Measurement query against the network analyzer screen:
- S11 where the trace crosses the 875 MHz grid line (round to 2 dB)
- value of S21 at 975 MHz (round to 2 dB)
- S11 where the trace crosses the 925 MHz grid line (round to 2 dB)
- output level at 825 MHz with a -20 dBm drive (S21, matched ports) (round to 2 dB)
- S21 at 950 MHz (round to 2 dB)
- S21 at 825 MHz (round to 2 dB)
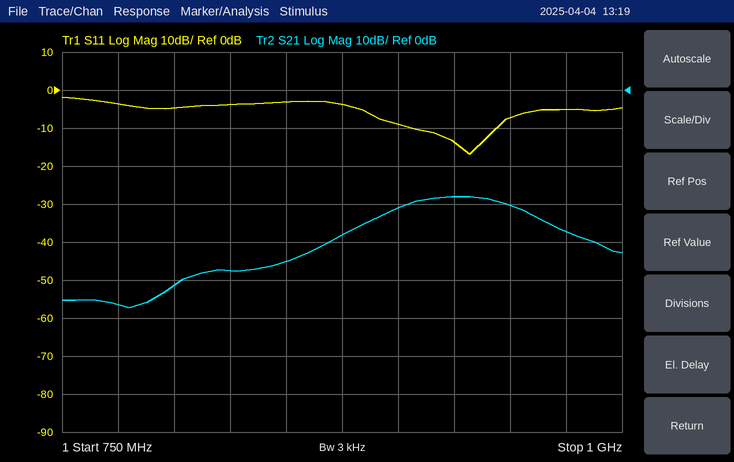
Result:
-4 dB
-38 dB
-14 dB
-68 dBm
-30 dB
-48 dB
